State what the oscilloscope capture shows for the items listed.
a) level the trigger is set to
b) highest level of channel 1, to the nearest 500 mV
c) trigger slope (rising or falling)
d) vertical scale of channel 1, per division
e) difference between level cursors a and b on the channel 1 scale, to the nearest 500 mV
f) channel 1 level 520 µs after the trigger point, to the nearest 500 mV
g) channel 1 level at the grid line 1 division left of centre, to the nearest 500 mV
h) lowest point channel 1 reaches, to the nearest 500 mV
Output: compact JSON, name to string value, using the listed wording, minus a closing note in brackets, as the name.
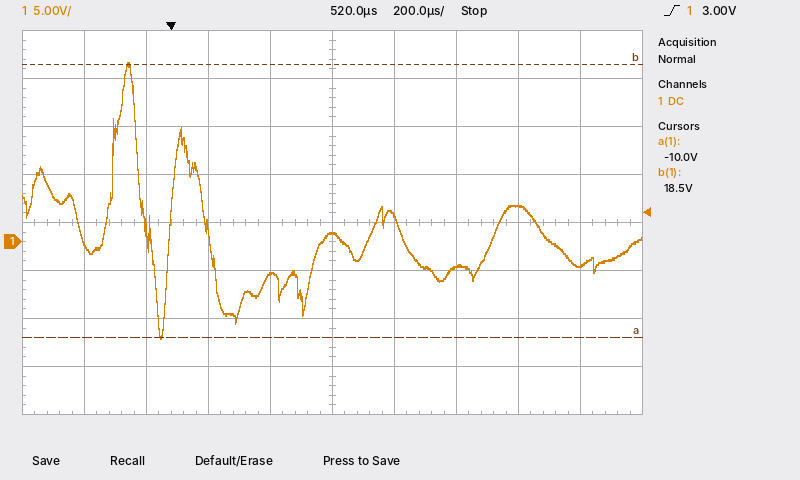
{"level the trigger is set to": "3.00 V", "highest level of channel 1, to the nearest 500 mV": "18.5 V", "trigger slope": "rising", "vertical scale of channel 1, per division": "5 V", "difference between level cursors a and b on the channel 1 scale, to the nearest 500 mV": "28.5 V", "channel 1 level 520 µs after the trigger point, to the nearest 500 mV": "1.0 V", "channel 1 level at the grid line 1 division left of centre, to the nearest 500 mV": "-3.5 V", "lowest point channel 1 reaches, to the nearest 500 mV": "-10.0 V"}
